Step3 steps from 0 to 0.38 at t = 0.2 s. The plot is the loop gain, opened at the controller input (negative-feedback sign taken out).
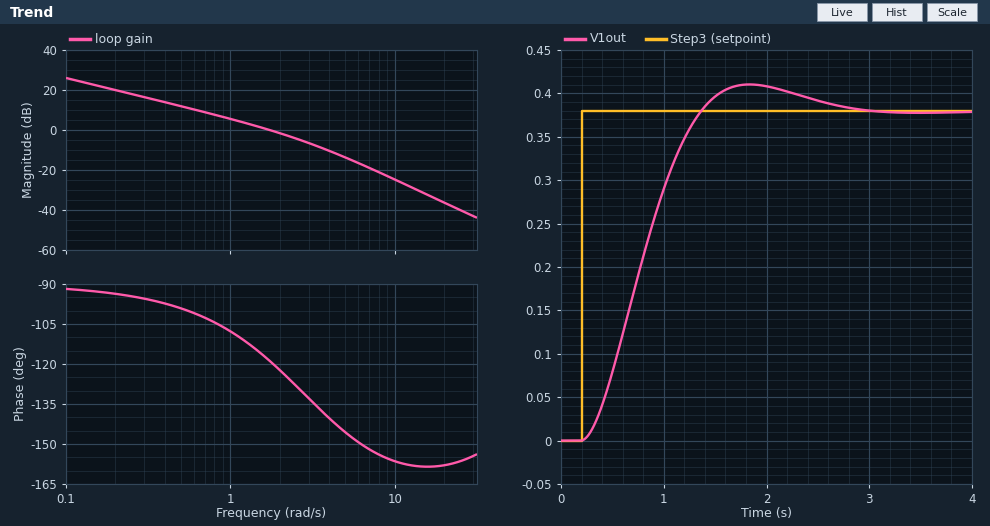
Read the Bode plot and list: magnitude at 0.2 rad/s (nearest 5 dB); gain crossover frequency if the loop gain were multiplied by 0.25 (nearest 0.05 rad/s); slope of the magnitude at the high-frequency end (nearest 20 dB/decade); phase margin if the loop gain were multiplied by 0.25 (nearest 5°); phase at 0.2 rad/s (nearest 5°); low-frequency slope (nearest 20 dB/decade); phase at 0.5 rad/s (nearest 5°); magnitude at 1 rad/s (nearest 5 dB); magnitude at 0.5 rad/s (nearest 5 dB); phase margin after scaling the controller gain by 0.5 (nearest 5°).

20 dB
0.50 rad/s
-40 dB/decade
80°
-95°
-20 dB/decade
-100°
5 dB
10 dB
75°
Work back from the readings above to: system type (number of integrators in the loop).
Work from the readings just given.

1
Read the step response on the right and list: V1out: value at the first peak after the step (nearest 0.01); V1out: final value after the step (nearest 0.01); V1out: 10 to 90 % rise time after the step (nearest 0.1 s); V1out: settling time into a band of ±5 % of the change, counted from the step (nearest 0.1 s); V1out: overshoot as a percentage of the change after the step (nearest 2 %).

0.41
0.38
0.8 s
2.1 s
8 %
